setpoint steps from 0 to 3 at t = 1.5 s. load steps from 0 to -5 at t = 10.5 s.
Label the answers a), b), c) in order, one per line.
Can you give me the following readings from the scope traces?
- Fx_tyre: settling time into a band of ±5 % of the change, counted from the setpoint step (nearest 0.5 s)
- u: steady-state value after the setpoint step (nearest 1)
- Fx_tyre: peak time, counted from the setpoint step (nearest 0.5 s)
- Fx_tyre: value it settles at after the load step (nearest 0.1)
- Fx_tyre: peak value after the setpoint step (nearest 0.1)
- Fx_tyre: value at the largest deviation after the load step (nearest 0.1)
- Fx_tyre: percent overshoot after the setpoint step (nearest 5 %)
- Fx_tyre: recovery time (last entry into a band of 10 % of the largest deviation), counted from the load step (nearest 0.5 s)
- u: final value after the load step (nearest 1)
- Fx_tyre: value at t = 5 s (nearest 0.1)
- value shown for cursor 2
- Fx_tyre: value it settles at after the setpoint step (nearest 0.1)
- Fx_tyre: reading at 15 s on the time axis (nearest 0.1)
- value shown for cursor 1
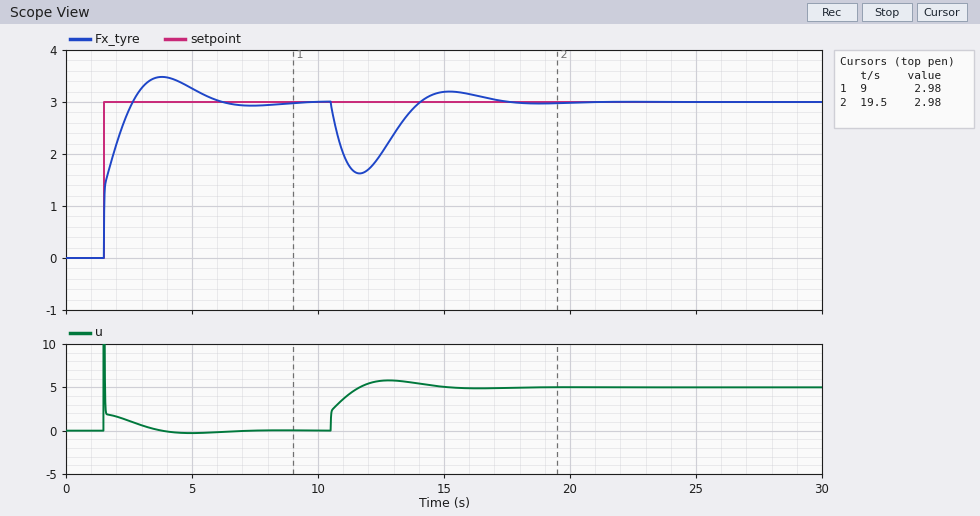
a) 4.0 s
b) 0
c) 2.5 s
d) 3.0
e) 3.5
f) 1.6
g) 15 %
h) 5.5 s
i) 5
j) 3.3
k) 2.98
l) 3.0
m) 3.2
n) 2.98
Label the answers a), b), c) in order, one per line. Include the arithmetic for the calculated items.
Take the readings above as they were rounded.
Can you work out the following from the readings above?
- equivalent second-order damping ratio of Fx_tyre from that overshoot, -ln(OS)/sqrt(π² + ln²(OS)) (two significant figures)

a) ln(0.15) = -1.897; 1.897 / sqrt(9.870 + 3.599) = 0.52
